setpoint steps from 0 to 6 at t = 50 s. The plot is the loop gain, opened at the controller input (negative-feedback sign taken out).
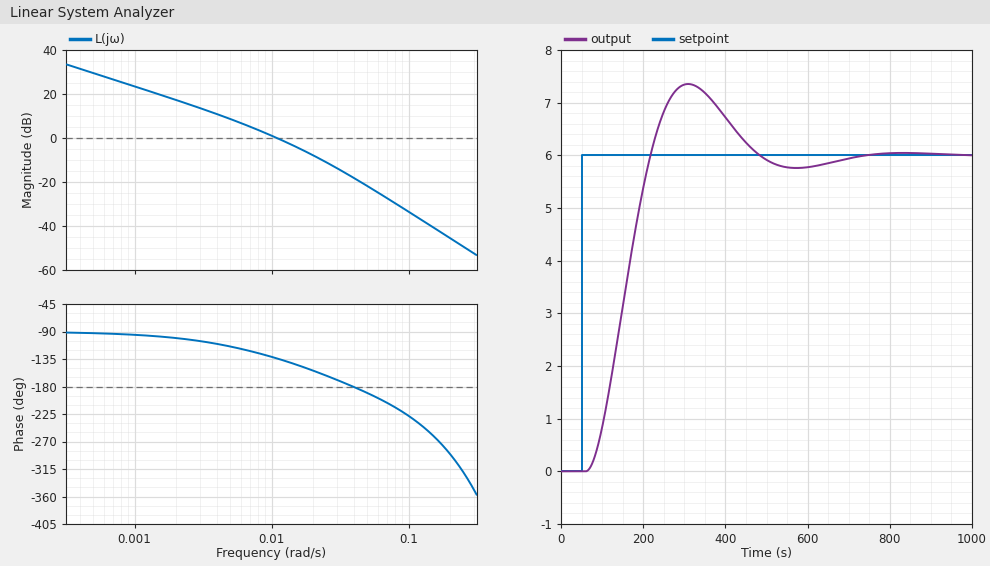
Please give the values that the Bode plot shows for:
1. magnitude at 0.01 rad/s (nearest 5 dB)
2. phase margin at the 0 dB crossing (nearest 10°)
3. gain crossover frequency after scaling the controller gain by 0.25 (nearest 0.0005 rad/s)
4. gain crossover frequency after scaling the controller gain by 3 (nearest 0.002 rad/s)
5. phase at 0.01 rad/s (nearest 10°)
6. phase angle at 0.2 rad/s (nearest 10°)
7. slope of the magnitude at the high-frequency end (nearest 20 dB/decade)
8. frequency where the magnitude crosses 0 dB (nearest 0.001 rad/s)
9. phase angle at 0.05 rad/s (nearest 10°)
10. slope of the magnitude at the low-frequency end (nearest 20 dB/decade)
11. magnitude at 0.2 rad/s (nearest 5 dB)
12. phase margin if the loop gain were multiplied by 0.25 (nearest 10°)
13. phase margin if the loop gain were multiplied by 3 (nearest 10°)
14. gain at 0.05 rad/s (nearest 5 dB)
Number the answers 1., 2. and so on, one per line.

1. 0 dB
2. 50°
3. 0.0035 rad/s
4. 0.022 rad/s
5. -130°
6. -290°
7. -40 dB/decade
8. 0.011 rad/s
9. -190°
10. -20 dB/decade
11. -45 dB
12. 70°
13. 20°
14. -20 dB
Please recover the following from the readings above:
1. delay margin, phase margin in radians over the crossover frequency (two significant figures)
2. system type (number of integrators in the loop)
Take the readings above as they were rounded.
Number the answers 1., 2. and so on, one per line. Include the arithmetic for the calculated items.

1. 50 × π / 180 / 0.011 = 79 s
2. 1
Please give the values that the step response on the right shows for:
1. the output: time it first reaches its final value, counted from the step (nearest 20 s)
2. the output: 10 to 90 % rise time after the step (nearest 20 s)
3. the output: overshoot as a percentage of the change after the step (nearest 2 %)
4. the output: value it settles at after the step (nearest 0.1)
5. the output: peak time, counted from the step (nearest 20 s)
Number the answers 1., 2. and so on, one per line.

1. 160 s
2. 100 s
3. 22 %
4. 6.0
5. 260 s
